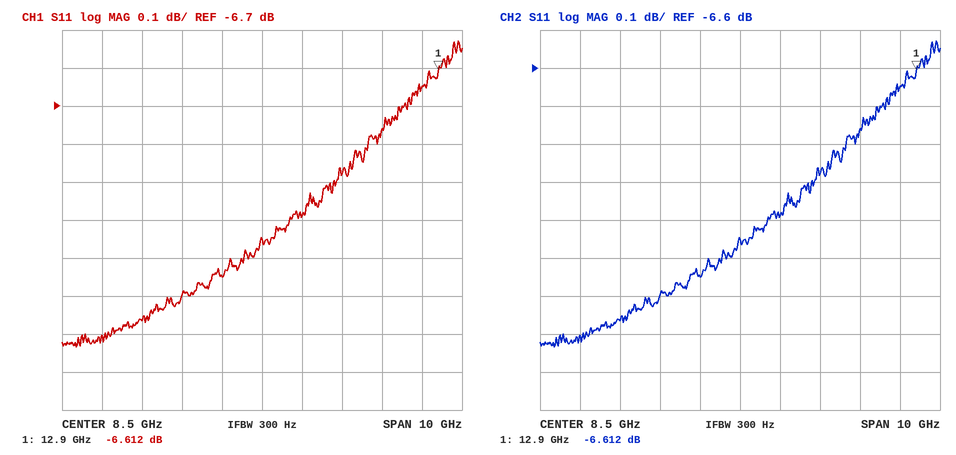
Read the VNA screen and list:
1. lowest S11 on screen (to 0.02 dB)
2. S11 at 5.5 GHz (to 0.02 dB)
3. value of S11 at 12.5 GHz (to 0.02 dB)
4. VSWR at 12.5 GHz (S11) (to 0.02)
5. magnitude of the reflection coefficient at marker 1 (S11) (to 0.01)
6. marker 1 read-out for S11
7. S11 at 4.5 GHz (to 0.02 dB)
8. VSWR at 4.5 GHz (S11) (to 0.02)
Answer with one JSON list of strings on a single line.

["-7.34 dB", "-7.26 dB", "-6.64 dB", "2.74", "0.47", "-6.612 dB", "-7.30 dB", "2.52"]
